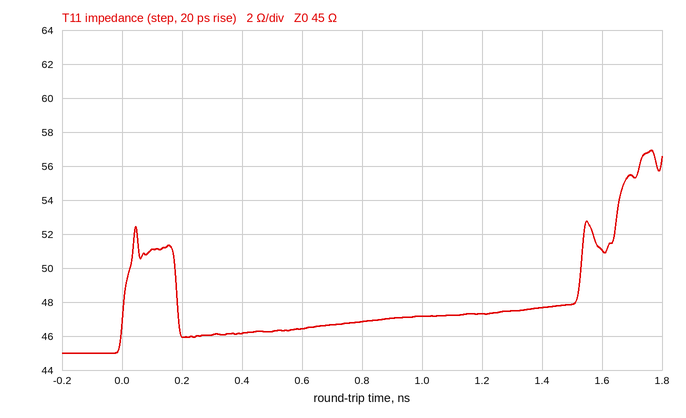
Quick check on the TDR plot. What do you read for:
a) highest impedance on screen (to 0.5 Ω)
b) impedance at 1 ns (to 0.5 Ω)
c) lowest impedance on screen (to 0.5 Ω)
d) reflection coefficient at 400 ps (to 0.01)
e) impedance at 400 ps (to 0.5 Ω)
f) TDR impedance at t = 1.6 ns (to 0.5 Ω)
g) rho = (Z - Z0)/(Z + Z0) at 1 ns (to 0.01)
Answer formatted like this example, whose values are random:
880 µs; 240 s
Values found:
57.0 Ω; 47.0 Ω; 45.0 Ω; +0.01; 46.0 Ω; 51.0 Ω; +0.02
